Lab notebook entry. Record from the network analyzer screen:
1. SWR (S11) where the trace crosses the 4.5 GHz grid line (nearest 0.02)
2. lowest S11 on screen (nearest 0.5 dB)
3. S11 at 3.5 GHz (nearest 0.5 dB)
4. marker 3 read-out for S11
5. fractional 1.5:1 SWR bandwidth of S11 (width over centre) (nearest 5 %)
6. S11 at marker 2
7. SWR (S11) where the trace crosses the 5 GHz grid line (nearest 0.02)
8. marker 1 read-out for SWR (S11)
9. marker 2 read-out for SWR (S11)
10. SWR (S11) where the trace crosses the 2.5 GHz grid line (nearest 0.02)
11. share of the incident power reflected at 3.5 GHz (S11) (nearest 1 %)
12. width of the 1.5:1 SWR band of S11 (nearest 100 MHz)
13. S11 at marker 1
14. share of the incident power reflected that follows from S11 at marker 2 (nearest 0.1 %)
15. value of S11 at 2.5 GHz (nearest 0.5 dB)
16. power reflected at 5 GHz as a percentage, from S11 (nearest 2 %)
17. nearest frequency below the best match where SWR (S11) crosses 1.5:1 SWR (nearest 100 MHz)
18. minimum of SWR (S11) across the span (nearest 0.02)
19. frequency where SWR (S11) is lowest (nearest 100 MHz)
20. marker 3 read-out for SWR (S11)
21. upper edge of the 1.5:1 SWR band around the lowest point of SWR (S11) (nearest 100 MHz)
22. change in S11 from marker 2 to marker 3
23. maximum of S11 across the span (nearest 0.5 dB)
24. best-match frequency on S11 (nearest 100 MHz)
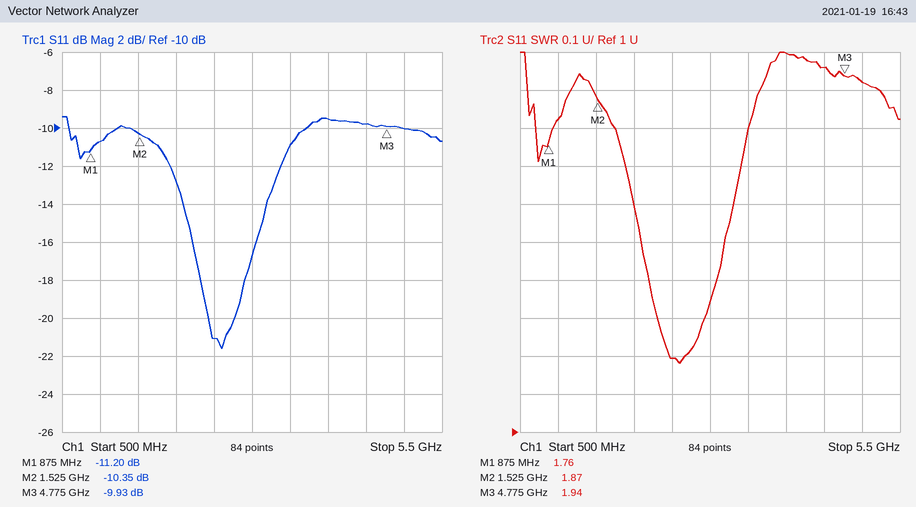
1.96
-21.5 dB
-11.0 dB
-9.93 dB
40 %
-10.35 dB
1.92
1.76
1.87
1.20
8 %
1.1 GHz
-11.20 dB
9.2 %
-21.0 dB
10 %
2.1 GHz
1.18
2.6 GHz
1.94
3.2 GHz
0.42 dB
-9.5 dB
2.6 GHz
